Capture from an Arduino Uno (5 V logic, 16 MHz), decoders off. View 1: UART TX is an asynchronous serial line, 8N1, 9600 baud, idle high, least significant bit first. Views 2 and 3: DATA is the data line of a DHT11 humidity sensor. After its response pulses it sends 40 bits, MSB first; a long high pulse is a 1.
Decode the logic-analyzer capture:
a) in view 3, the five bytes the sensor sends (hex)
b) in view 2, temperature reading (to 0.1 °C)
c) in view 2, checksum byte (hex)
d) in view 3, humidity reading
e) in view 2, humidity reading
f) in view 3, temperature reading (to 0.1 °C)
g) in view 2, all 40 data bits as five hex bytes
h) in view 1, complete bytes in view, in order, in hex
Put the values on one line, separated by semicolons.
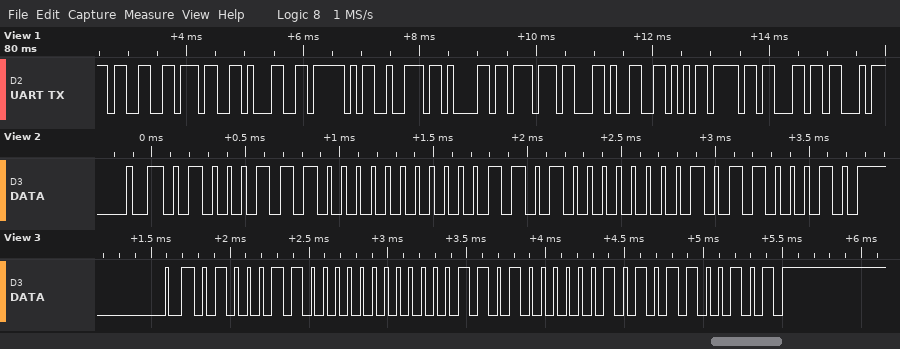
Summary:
46 00 1A 05 65; 26.1 °C; 0x62; 70 %; 71 %; 26.5 °C; 47 00 1A 01 62; 33 37 31 5F 72 61 77 2C 56 6F 6C
